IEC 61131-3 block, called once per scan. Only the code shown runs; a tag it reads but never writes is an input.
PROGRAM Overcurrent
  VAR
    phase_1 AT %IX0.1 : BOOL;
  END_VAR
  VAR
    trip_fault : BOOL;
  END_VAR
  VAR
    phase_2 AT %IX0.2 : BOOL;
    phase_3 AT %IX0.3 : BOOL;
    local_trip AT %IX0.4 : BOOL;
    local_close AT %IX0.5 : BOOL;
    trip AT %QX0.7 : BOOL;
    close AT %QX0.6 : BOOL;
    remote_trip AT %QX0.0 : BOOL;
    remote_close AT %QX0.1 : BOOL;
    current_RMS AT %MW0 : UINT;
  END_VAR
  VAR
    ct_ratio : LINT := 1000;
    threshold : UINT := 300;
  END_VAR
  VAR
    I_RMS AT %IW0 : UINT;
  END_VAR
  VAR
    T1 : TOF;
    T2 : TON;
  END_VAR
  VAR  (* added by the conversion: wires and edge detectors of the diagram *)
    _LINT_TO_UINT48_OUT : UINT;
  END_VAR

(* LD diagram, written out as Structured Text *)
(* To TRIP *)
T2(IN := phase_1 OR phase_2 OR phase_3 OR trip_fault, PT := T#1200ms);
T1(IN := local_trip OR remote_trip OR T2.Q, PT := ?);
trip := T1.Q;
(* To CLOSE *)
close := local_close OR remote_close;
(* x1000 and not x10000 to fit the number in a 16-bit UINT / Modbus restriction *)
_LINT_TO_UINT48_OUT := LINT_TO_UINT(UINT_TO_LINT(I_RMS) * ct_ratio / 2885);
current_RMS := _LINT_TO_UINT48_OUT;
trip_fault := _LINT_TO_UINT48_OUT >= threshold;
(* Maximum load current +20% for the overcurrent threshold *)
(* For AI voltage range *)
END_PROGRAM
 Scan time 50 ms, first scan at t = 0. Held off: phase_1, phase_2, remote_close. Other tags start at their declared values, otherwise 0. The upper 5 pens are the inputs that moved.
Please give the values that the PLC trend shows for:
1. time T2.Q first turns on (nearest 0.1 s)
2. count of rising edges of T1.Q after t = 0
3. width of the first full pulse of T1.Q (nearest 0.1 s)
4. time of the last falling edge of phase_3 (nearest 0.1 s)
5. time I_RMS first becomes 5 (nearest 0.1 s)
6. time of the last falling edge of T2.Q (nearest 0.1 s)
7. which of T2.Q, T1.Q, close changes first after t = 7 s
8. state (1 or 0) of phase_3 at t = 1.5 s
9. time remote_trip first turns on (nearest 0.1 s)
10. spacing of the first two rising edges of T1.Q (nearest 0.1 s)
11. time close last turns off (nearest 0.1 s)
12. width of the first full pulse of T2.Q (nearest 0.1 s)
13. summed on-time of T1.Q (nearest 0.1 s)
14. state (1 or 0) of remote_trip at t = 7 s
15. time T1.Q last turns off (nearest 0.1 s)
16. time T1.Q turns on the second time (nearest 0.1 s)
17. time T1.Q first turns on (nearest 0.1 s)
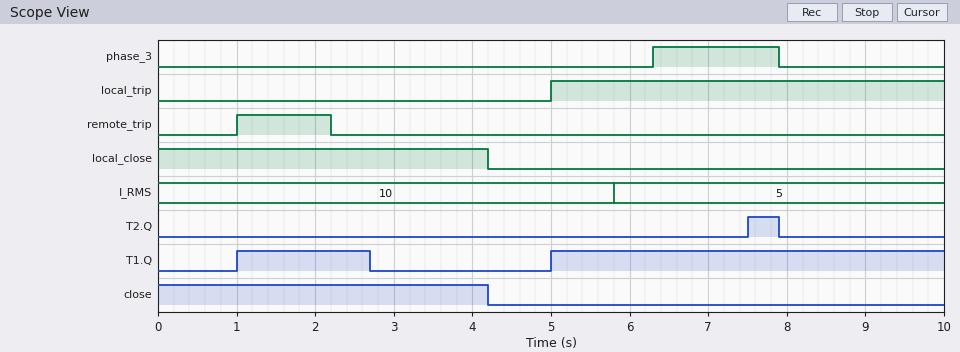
7.5 s
2
1.7 s
7.9 s
5.8 s
7.9 s
T2.Q
0
1.0 s
4.0 s
4.2 s
0.4 s
6.7 s
0
2.7 s
5.0 s
1.0 s
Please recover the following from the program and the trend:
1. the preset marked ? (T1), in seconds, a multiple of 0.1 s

0.5 s
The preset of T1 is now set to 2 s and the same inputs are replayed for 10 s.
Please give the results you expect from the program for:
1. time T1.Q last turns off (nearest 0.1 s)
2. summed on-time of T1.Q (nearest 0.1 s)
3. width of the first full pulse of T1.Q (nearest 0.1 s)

4.2 s
8.2 s
3.2 s
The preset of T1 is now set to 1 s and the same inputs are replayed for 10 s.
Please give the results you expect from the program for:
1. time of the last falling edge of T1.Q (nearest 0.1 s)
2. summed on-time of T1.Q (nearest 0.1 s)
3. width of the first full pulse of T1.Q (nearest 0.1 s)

3.2 s
7.2 s
2.2 s
